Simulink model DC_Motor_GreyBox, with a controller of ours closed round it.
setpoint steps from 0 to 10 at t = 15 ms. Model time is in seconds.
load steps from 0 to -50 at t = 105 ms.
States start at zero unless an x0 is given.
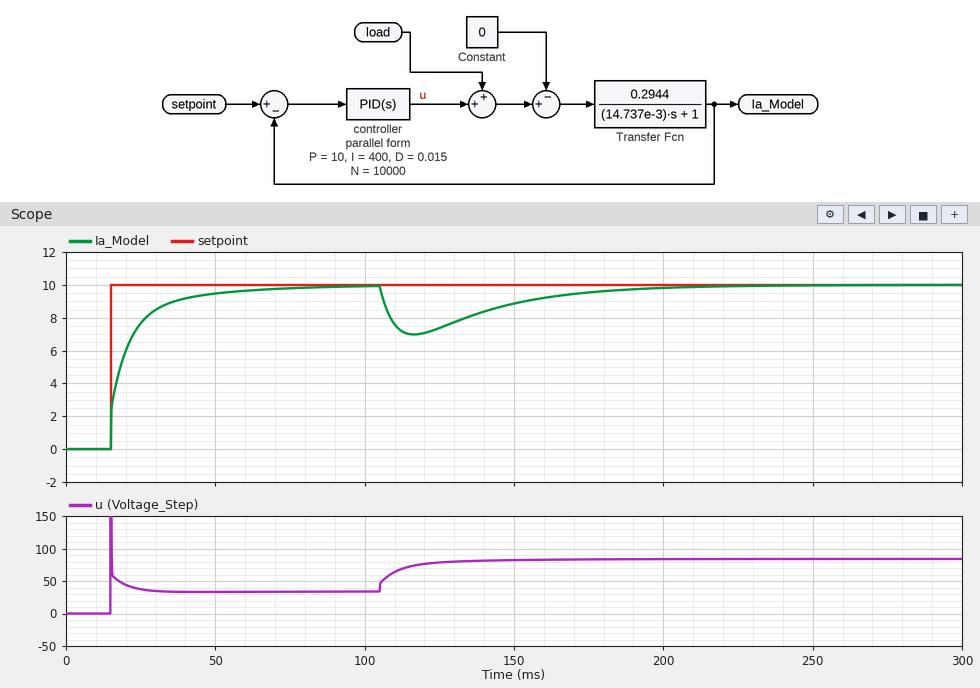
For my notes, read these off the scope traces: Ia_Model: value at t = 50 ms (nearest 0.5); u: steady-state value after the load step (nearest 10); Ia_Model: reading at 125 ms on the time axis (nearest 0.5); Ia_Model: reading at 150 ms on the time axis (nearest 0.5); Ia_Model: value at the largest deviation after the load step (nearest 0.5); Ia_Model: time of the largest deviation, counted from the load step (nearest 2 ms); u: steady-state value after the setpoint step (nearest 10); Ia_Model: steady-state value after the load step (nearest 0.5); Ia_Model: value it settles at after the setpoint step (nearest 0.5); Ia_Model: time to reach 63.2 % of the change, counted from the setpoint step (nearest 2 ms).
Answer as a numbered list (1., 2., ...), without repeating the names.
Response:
1. 9.5
2. 80
3. 7.5
4. 9.0
5. 7.0
6. 12 ms
7. 30
8. 10.0
9. 10.0
10. 6 ms
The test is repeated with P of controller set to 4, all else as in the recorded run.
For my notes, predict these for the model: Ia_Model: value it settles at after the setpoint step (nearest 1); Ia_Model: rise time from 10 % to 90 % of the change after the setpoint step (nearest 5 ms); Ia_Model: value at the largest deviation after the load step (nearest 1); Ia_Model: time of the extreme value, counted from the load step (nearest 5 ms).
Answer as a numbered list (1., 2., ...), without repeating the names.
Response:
1. 10
2. 25 ms
3. 6
4. 15 ms
